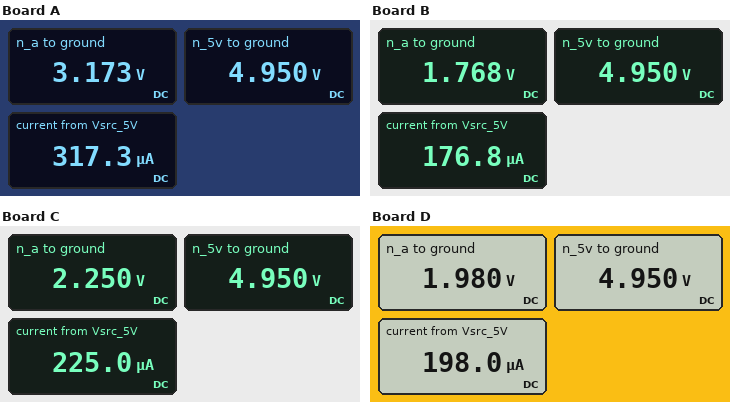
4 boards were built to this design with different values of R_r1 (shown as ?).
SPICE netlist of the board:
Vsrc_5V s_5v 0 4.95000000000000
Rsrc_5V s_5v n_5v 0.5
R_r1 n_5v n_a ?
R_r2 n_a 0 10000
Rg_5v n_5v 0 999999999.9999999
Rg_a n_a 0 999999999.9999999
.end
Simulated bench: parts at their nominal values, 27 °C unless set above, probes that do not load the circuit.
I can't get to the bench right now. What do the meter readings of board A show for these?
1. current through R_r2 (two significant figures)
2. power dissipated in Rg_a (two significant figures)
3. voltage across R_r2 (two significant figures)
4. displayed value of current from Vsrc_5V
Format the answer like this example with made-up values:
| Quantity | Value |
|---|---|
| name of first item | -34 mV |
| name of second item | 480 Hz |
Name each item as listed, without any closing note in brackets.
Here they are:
| Quantity | Value |
|---|---|
| current through R_r2 | 320 µA |
| power dissipated in Rg_a | 10 nW |
| voltage across R_r2 | 3.2 V |
| displayed value of current from Vsrc_5V | 317.3 µA |
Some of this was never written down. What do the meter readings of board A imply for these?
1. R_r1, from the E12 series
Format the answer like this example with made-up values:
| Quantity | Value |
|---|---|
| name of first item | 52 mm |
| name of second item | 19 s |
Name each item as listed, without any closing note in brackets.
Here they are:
| Quantity | Value |
|---|---|
| R_r1, from the E12 series | 5.6 kΩ |
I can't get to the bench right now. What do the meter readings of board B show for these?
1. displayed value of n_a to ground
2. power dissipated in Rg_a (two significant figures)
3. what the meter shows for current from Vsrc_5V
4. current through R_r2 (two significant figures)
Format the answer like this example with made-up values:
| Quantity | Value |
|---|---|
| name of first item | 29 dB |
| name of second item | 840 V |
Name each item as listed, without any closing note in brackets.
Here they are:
| Quantity | Value |
|---|---|
| displayed value of n_a to ground | 1.768 V |
| power dissipated in Rg_a | 3.1 nW |
| what the meter shows for current from Vsrc_5V | 176.8 µA |
| current through R_r2 | 180 µA |
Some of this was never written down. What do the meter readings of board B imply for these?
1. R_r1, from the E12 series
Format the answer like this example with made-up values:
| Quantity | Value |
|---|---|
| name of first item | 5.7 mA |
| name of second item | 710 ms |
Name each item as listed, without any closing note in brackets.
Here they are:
| Quantity | Value |
|---|---|
| R_r1, from the E12 series | 18 kΩ |
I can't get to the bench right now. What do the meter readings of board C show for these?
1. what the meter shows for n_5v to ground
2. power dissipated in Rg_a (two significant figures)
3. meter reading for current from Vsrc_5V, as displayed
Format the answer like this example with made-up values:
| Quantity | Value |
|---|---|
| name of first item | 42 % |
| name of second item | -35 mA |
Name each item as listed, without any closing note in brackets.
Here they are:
| Quantity | Value |
|---|---|
| what the meter shows for n_5v to ground | 4.950 V |
| power dissipated in Rg_a | 5.1 nW |
| meter reading for current from Vsrc_5V, as displayed | 225.0 µA |
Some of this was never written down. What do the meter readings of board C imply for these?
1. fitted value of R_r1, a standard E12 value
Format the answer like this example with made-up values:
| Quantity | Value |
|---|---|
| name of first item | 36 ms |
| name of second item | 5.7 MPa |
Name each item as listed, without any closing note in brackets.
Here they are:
| Quantity | Value |
|---|---|
| fitted value of R_r1, a standard E12 value | 12 kΩ |
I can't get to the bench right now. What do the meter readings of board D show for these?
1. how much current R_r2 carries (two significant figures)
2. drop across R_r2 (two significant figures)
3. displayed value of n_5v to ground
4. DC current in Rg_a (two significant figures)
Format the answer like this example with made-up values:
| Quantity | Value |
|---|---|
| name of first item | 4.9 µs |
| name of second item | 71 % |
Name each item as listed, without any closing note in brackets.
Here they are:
| Quantity | Value |
|---|---|
| how much current R_r2 carries | 200 µA |
| drop across R_r2 | 2.0 V |
| displayed value of n_5v to ground | 4.950 V |
| DC current in Rg_a | 2.0 nA |
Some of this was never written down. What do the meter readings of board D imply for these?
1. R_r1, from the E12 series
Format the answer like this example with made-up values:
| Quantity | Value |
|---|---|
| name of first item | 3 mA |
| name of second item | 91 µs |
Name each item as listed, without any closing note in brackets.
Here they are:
| Quantity | Value |
|---|---|
| R_r1, from the E12 series | 15 kΩ |
